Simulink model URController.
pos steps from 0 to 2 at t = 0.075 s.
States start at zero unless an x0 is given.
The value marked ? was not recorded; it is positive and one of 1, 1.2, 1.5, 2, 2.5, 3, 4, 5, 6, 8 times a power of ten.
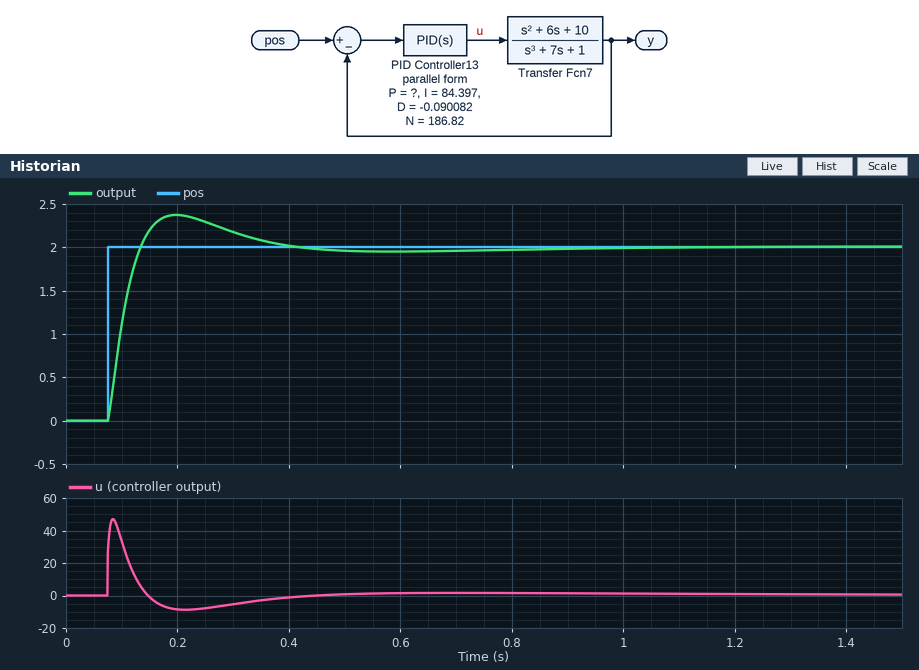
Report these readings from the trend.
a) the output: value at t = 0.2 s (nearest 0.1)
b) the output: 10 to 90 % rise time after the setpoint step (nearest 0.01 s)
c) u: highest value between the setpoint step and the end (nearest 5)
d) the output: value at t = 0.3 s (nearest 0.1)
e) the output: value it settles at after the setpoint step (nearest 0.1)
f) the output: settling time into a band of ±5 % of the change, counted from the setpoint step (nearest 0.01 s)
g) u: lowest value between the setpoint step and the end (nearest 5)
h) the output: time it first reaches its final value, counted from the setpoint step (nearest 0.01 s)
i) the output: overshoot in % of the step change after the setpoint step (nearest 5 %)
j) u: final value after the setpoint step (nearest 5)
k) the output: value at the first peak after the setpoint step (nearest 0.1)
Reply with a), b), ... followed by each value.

a) 2.4
b) 0.04 s
c) 45
d) 2.2
e) 2.0
f) 0.26 s
g) -10
h) 0.06 s
i) 20 %
j) 0
k) 2.4
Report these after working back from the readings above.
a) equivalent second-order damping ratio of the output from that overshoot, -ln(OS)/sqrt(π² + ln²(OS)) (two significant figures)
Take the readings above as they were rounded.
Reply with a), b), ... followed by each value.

a) 0.46
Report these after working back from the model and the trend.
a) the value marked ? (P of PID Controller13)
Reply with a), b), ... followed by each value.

a) 30
